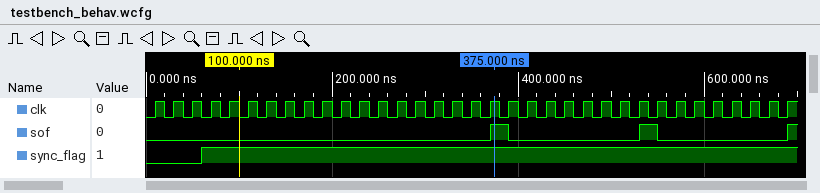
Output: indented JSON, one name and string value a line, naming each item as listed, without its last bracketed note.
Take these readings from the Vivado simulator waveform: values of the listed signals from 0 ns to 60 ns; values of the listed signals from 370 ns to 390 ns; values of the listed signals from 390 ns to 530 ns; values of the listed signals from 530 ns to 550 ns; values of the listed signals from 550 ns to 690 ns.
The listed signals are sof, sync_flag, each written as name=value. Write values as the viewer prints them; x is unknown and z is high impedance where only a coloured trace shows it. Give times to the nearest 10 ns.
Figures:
{
  "values of the listed signals from 0 ns to 60 ns": "sof=0, sync_flag=0",
  "values of the listed signals from 370 ns to 390 ns": "sof=1, sync_flag=1",
  "values of the listed signals from 390 ns to 530 ns": "sof=0, sync_flag=1",
  "values of the listed signals from 530 ns to 550 ns": "sof=1, sync_flag=1",
  "values of the listed signals from 550 ns to 690 ns": "sof=0, sync_flag=1"
}
